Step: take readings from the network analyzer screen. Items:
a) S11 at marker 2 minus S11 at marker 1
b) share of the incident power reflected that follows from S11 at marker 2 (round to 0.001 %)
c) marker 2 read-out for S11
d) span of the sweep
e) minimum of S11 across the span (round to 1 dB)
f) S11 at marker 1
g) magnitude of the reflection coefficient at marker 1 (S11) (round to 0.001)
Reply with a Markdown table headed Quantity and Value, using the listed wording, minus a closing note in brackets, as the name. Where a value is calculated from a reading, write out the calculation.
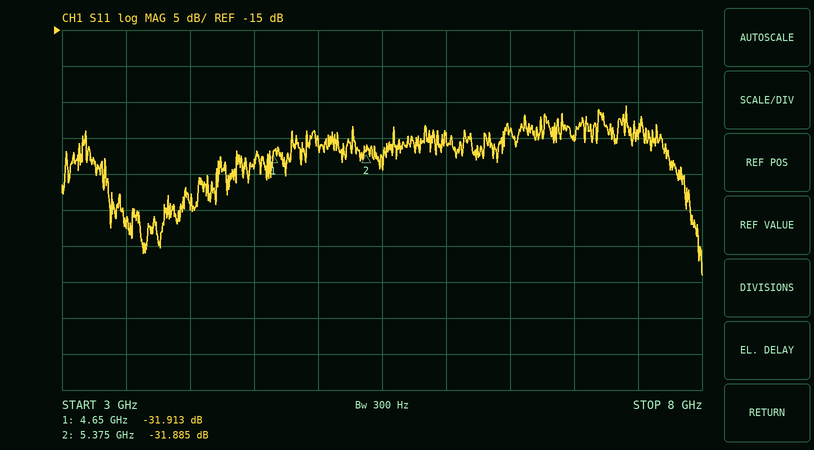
| Quantity | Value |
|---|---|
| S11 at marker 2 minus S11 at marker 1 | -31.885 − (-31.913) = 0.028 dB |
| share of the incident power reflected that follows from S11 at marker 2 | 10^(-31.885/10) ≈ 0.065 % |
| marker 2 read-out for S11 | -31.885 dB |
| span of the sweep | 5 GHz |
| minimum of S11 across the span | -49 dB |
| S11 at marker 1 | -31.913 dB |
| magnitude of the reflection coefficient at marker 1 (S11) | 10^(-31.913/20) ≈ 0.025 |
